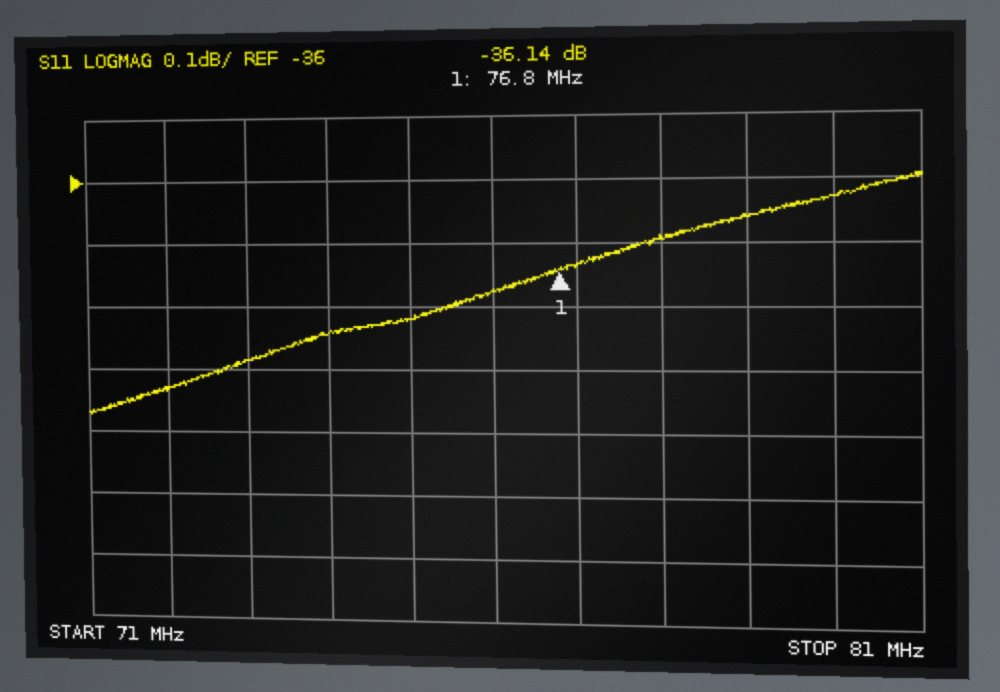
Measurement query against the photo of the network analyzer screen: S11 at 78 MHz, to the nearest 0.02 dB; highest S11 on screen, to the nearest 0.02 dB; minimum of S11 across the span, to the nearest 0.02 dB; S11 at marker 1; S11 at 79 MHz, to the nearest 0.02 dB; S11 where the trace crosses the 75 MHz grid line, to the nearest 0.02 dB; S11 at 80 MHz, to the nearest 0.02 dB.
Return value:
-36.10 dB
-36.00 dB
-36.38 dB
-36.14 dB
-36.06 dB
-36.22 dB
-36.02 dB
